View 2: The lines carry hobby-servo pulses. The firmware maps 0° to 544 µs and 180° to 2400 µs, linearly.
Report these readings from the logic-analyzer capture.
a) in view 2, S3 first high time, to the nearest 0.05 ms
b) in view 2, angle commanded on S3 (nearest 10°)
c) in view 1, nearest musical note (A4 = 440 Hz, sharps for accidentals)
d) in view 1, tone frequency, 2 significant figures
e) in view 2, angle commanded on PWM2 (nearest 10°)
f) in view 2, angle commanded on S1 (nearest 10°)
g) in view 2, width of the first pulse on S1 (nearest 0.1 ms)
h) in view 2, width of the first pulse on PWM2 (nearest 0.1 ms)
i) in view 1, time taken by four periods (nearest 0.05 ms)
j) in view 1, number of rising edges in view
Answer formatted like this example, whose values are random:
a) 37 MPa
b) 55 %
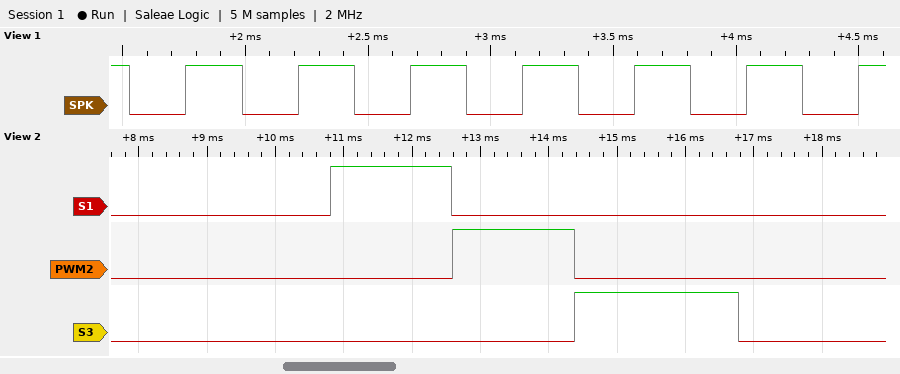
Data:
a) 2.40 ms
b) 180°
c) C#7
d) 2.2 kHz
e) 120°
f) 120°
g) 1.8 ms
h) 1.8 ms
i) 1.80 ms
j) 7
